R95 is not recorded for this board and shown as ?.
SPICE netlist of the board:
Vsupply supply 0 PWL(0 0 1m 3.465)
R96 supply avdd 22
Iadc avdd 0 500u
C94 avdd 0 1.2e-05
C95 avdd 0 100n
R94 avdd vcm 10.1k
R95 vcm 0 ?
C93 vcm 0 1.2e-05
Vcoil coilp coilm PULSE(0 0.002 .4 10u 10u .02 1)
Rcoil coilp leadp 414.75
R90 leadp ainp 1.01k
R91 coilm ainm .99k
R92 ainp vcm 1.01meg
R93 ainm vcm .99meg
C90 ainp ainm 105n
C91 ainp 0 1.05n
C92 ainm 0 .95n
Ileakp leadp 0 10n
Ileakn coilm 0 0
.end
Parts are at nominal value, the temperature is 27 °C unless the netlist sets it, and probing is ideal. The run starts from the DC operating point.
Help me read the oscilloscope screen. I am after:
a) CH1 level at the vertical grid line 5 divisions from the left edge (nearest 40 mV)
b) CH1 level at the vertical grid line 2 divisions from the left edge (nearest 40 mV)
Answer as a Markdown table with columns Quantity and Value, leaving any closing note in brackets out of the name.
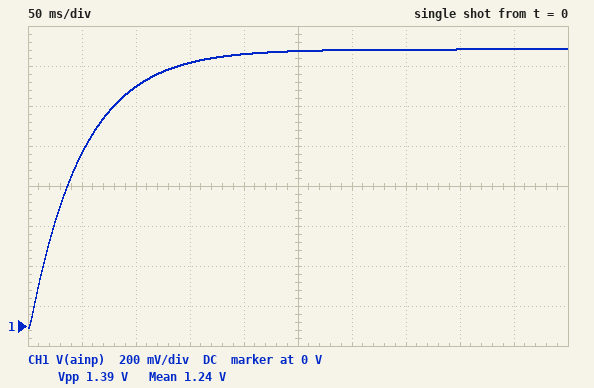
| Quantity | Value |
|---|---|
| CH1 level at the vertical grid line 5 divisions from the left edge | 1.36 V |
| CH1 level at the vertical grid line 2 divisions from the left edge | 1.20 V |
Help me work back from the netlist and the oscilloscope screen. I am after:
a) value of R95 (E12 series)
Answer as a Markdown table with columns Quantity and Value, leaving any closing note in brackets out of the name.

| Quantity | Value |
|---|---|
| value of R95 | 6.8 kΩ |
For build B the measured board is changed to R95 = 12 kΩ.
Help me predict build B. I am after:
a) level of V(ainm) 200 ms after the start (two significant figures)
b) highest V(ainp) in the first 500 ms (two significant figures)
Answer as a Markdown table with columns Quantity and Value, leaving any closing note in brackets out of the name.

| Quantity | Value |
|---|---|
| level of V(ainm) 200 ms after the start | 1.8 V |
| highest V(ainp) in the first 500 ms | 1.9 V |
